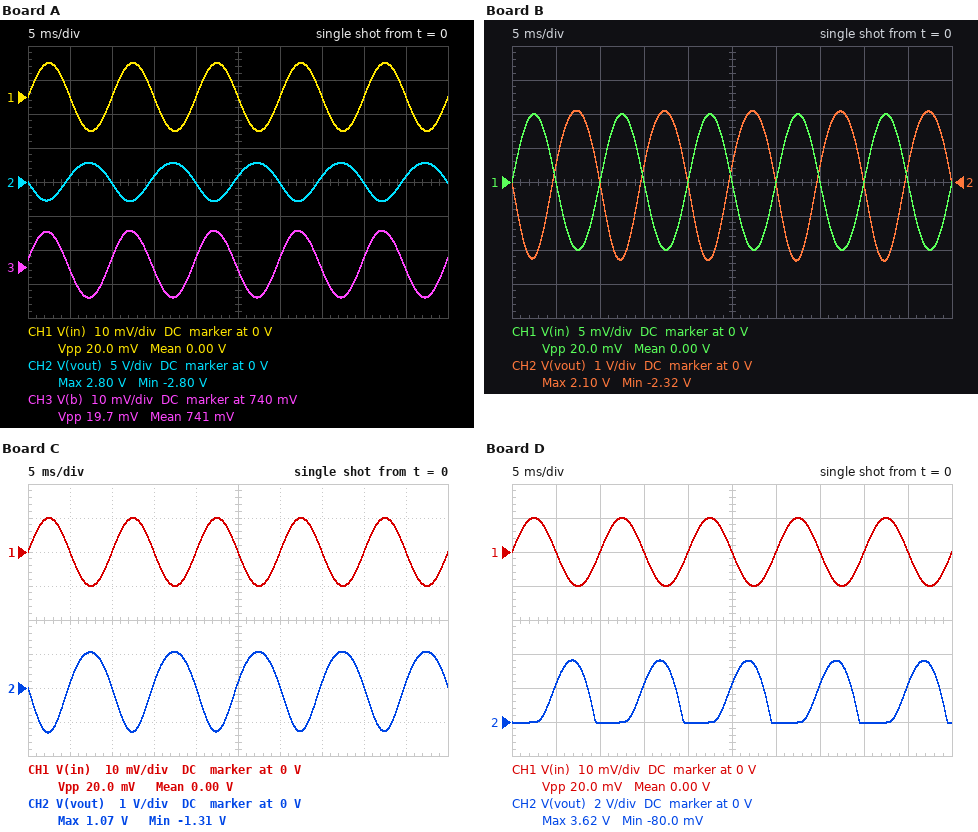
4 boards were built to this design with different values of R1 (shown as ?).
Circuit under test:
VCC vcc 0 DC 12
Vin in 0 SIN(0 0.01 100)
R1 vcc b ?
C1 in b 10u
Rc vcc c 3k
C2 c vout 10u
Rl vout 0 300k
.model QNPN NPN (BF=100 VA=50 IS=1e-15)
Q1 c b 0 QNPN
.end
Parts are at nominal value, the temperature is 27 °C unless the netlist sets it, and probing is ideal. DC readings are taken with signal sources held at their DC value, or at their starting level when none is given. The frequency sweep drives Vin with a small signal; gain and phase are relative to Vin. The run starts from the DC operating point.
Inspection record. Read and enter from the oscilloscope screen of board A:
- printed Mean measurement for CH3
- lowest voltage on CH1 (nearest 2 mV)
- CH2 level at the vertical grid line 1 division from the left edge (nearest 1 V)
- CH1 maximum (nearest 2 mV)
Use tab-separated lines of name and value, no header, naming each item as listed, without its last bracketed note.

printed Mean measurement for CH3	741 mV
lowest voltage on CH1	-10 mV
CH2 level at the vertical grid line 1 division from the left edge	1 V
CH1 maximum	10 mV
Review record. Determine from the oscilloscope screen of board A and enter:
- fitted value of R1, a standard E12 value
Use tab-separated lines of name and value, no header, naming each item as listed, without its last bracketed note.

fitted value of R1, a standard E12 value	390 kΩ
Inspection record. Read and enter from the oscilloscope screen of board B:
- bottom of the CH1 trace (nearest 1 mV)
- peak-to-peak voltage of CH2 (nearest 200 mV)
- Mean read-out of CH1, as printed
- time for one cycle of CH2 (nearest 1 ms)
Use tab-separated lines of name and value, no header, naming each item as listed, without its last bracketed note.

bottom of the CH1 trace	-10 mV
peak-to-peak voltage of CH2	4.4 V
Mean read-out of CH1, as printed	0.00 V
time for one cycle of CH2	10 ms
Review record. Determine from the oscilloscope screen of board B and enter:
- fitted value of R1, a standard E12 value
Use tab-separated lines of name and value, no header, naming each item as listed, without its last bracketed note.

fitted value of R1, a standard E12 value	560 kΩ
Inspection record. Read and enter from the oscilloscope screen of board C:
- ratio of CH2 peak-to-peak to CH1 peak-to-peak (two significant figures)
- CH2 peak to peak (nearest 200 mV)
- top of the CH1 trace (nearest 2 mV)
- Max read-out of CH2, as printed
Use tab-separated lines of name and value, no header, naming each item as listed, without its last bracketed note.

ratio of CH2 peak-to-peak to CH1 peak-to-peak	120
CH2 peak to peak	2.4 V
top of the CH1 trace	10 mV
Max read-out of CH2, as printed	1.07 V
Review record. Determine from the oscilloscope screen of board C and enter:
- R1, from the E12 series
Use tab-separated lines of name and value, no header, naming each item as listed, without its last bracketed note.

R1, from the E12 series	1.2 MΩ
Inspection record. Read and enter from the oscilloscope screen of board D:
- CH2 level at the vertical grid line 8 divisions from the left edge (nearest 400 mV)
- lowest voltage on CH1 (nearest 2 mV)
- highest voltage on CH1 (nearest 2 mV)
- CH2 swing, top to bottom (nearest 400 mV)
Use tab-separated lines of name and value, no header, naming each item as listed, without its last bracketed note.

CH2 level at the vertical grid line 8 divisions from the left edge	0 V
lowest voltage on CH1	-10 mV
highest voltage on CH1	10 mV
CH2 swing, top to bottom	3.6 V
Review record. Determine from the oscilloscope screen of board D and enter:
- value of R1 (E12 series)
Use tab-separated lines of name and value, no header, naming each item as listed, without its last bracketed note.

value of R1	220 kΩ
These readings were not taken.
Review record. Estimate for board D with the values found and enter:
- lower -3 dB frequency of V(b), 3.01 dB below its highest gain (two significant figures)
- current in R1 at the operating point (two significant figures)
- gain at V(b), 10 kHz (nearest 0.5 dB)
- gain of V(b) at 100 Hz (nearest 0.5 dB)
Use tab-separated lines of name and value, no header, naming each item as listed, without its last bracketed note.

lower -3 dB frequency of V(b), 3.01 dB below its highest gain	850 Hz
current in R1 at the operating point	51 µA
gain at V(b), 10 kHz	0 dB
gain of V(b) at 100 Hz	-18.5 dB
